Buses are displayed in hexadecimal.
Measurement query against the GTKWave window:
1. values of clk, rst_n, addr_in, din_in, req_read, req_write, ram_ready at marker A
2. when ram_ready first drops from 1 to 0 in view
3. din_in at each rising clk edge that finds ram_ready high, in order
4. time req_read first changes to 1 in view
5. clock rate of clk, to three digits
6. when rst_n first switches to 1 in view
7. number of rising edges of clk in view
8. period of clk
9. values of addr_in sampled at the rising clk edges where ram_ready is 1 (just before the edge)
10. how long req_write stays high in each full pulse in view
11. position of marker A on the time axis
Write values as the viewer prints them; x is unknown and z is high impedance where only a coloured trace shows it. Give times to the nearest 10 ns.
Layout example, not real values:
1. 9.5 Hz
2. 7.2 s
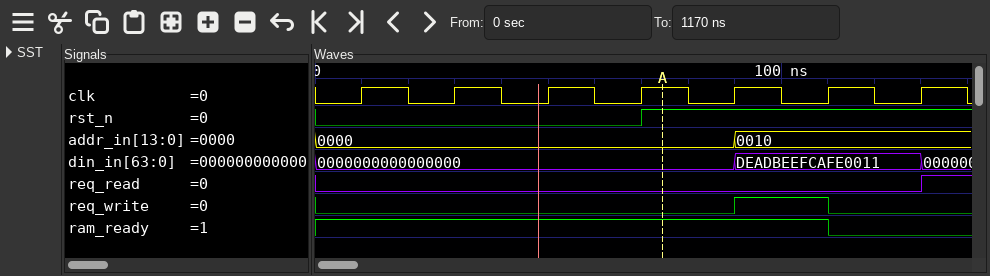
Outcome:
1. clk=1, rst_n=1, addr_in=0000, din_in=0000000000000000, req_read=0, req_write=0, ram_ready=1
2. 110 ns
3. 0000000000000000, 0000000000000000, 0000000000000000, 0000000000000000, 0000000000000000, DEADBEEFCAFE0011
4. 130 ns
5. 50.0 MHz
6. 70 ns
7. 7
8. 20 ns
9. 0000, 0000, 0000, 0000, 0000, 0010
10. 20 ns
11. 70 ns
